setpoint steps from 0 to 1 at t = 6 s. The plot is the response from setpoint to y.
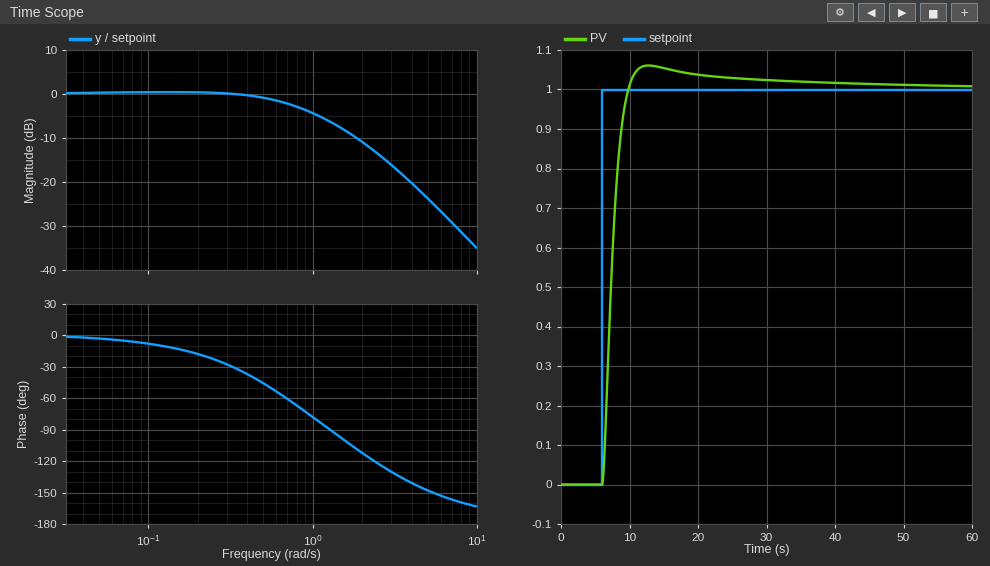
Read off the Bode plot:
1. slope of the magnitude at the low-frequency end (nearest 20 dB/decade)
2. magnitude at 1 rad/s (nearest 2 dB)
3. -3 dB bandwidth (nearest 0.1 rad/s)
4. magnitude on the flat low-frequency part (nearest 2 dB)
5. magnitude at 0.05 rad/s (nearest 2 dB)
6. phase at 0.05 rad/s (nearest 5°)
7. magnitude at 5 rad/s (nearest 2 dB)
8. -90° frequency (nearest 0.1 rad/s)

0 dB/decade
-4 dB
0.8 rad/s
0 dB
0 dB
-5°
-24 dB
1.3 rad/s
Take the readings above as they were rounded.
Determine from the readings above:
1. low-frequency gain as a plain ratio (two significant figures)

1.0
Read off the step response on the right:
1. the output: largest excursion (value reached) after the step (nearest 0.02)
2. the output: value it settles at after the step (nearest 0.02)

1.06
1.00
